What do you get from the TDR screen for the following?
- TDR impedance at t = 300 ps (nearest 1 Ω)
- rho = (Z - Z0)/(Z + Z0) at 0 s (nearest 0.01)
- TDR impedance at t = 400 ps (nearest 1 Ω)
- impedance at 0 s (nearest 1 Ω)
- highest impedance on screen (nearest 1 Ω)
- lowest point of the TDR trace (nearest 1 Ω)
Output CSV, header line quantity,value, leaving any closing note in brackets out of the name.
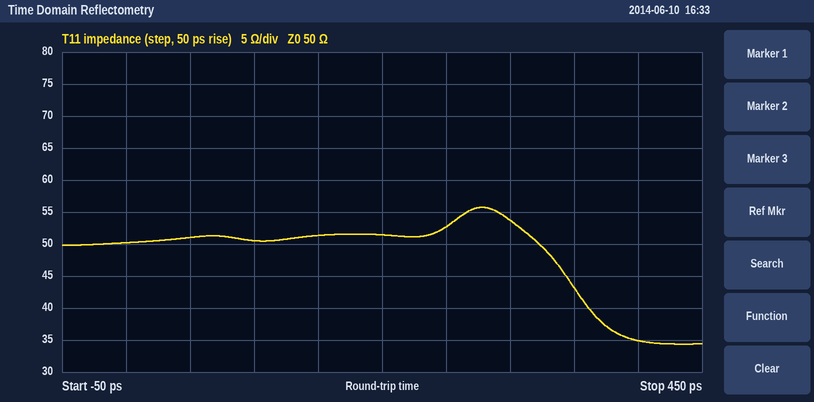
quantity,value
TDR impedance at t = 300 ps,54 Ω
rho = (Z - Z0)/(Z + Z0) at 0 s,0.00
TDR impedance at t = 400 ps,35 Ω
impedance at 0 s,50 Ω
highest impedance on screen,56 Ω
lowest point of the TDR trace,34 Ω
